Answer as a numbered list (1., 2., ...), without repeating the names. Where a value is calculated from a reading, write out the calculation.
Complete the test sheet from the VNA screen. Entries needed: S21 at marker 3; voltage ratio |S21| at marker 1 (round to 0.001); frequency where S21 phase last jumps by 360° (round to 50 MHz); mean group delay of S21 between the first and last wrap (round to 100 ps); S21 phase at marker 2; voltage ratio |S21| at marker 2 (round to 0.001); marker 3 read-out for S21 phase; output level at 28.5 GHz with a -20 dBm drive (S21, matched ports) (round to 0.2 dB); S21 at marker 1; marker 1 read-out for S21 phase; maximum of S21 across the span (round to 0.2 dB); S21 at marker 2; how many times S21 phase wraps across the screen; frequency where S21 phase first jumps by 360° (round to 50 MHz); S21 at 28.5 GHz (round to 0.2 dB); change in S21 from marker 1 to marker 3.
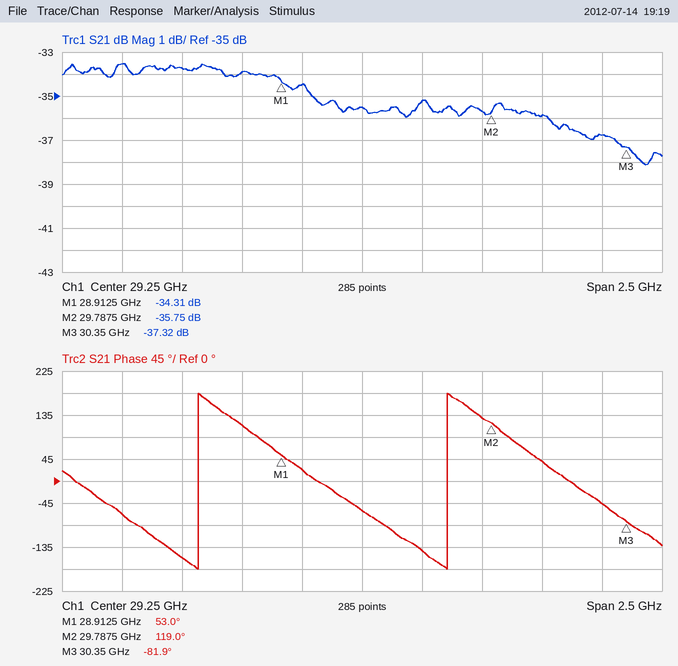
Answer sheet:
1. -37.32 dB
2. 10^(-34.31/20) ≈ 0.019
3. 29.60 GHz
4. 1 cycle / (29.60 GHz − 28.55 GHz) ≈ 1.0 ns
5. 119.0°
6. 10^(-35.75/20) ≈ 0.016
7. -81.9°
8. -20 dBm + (-33.8 dB) = -53.8 dBm
9. -34.31 dB
10. 53.0°
11. -33.6 dB
12. -35.75 dB
13. 2
14. 28.55 GHz
15. -33.8 dB
16. -37.32 − (-34.31) = -3.01 dB
